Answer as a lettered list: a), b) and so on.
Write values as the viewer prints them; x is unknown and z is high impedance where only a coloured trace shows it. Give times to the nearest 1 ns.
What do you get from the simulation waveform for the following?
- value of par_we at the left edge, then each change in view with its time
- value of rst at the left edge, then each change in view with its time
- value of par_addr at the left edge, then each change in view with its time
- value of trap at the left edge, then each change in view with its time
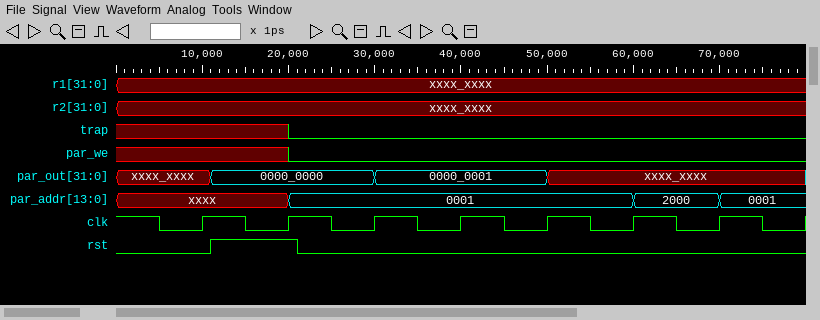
a) x, 0 at 20 ns
b) 0, 1 at 11 ns, 0 at 21 ns
c) xxxx, 0001 at 20 ns, 2000 at 60 ns, 0001 at 70 ns
d) x, 0 at 20 ns
